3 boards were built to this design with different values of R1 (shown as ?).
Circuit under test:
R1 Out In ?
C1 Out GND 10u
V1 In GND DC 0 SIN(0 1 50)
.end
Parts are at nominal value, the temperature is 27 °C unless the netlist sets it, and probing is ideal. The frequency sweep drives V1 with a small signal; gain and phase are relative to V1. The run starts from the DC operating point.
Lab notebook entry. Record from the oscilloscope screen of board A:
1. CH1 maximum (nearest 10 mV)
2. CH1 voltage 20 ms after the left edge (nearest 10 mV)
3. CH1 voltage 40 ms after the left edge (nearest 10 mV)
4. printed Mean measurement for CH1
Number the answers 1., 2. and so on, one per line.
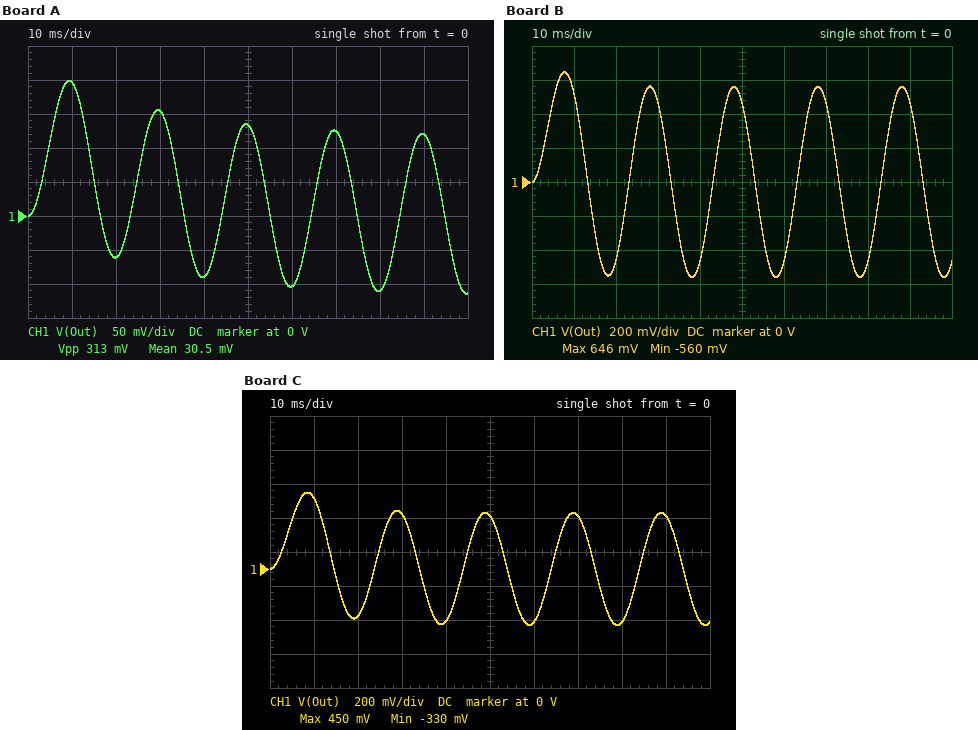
1. 200 mV
2. -60 mV
3. -90 mV
4. 30.5 mV
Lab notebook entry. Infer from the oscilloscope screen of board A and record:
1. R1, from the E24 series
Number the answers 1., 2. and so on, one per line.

1. 2.7 kΩ
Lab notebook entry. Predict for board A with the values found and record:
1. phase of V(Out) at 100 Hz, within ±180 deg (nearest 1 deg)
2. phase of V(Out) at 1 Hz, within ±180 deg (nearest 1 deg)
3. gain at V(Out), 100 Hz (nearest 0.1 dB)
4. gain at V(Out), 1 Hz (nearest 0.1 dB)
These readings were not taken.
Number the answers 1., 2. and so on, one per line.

1. -87 deg
2. -10 deg
3. -24.6 dB
4. -0.1 dB
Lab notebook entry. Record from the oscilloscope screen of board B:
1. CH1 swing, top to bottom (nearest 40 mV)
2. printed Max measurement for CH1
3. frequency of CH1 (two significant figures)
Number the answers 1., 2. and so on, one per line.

1. 1.20 V
2. 646 mV
3. 50 Hz
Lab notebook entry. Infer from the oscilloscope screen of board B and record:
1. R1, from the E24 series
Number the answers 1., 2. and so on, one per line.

1. 470 Ω
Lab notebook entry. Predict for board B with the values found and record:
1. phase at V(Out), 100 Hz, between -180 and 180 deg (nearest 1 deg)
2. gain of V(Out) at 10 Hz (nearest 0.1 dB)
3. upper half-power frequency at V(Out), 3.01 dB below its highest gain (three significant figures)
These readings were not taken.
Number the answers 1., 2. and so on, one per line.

1. -71 deg
2. -0.4 dB
3. 33.9 Hz
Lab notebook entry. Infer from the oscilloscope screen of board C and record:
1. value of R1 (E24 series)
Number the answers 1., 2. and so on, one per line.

1. 910 Ω
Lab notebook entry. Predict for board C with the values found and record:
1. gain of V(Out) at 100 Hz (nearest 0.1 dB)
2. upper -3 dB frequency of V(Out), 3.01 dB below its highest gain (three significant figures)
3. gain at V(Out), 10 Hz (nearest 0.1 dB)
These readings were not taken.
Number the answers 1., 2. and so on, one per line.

1. -15.3 dB
2. 17.5 Hz
3. -1.2 dB
